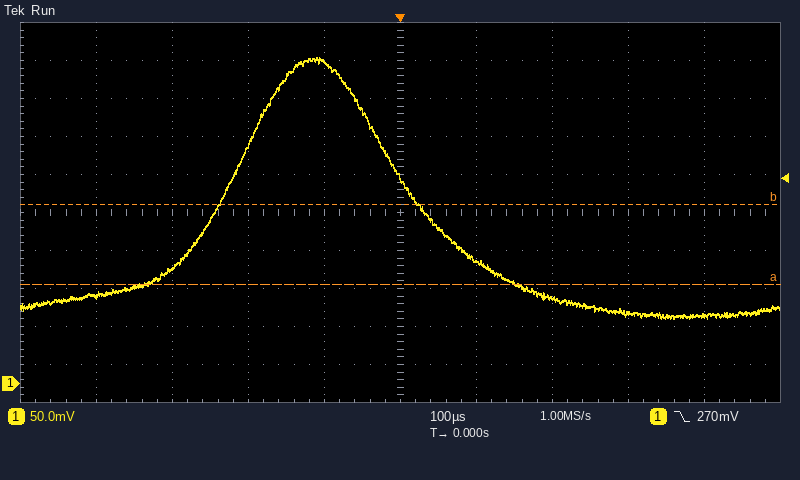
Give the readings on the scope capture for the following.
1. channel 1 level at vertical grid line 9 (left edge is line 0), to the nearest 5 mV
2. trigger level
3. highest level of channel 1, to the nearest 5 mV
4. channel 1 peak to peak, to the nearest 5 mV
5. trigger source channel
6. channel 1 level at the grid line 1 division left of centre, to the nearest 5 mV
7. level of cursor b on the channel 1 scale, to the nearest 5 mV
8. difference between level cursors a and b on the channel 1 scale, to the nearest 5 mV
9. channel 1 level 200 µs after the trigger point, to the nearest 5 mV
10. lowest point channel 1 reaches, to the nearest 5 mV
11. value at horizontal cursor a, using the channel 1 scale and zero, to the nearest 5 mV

90 mV
270 mV
430 mV
345 mV
channel 1
425 mV
235 mV
105 mV
110 mV
85 mV
130 mV
